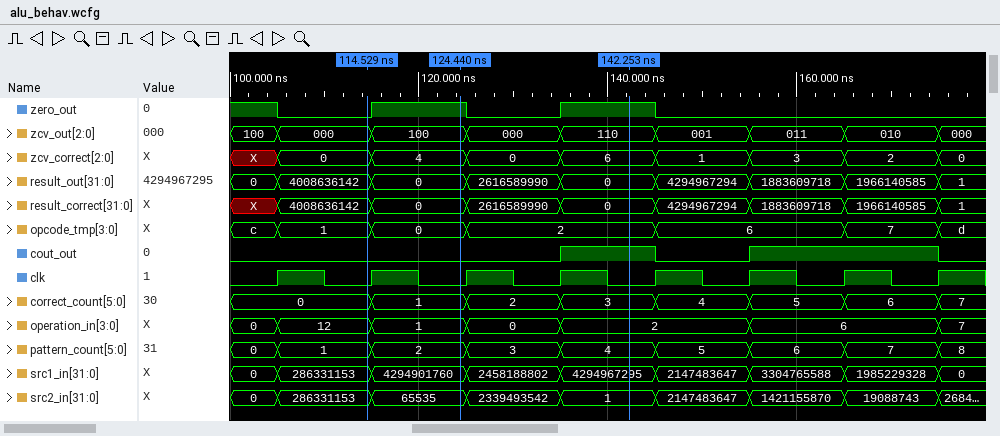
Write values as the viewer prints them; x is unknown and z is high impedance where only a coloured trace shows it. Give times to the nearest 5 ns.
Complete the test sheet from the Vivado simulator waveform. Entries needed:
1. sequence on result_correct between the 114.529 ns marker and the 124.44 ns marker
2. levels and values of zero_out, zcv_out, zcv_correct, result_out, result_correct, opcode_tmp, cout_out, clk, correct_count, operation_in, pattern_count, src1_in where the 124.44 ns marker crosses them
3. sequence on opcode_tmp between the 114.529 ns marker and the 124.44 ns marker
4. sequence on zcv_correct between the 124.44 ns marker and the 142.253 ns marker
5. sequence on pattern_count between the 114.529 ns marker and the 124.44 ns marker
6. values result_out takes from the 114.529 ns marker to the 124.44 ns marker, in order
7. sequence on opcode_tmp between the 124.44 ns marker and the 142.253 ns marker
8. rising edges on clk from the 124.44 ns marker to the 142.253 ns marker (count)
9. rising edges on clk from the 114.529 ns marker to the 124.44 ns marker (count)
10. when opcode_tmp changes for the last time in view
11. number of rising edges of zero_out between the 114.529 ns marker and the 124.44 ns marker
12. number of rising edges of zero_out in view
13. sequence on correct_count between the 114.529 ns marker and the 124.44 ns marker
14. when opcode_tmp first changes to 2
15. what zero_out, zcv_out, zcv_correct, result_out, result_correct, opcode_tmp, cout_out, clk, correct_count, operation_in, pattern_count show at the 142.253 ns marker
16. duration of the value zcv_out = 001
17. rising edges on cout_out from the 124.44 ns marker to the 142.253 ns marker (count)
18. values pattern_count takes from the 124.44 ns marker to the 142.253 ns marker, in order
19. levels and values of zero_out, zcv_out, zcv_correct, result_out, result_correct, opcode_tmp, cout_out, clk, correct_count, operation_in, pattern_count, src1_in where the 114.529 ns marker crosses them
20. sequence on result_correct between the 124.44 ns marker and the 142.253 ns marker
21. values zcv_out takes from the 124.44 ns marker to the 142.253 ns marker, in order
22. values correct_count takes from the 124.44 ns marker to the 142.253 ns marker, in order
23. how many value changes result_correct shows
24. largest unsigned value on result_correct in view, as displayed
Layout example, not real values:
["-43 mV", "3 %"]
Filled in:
["4008636142, 0", "zero_out=1, zcv_out=100, zcv_correct=4, result_out=0, result_correct=0, opcode_tmp=0, cout_out=0, clk=0, correct_count=1, operation_in=1, pattern_count=2, src1_in=4294901760", "1, 0", "4, 0, 6", "1, 2", "4008636142, 0", "0, 2", "2", "1", "175 ns", "1", "2", "0, 1", "125 ns", "zero_out=1, zcv_out=110, zcv_correct=6, result_out=0, result_correct=0, opcode_tmp=2, cout_out=1, clk=0, correct_count=3, operation_in=2, pattern_count=4", "10 ns", "1", "2, 3, 4", "zero_out=0, zcv_out=000, zcv_correct=0, result_out=4008636142, result_correct=4008636142, opcode_tmp=1, cout_out=0, clk=0, correct_count=0, operation_in=12, pattern_count=1, src1_in=286331153", "0, 2616589990, 0", "100, 000, 110", "1, 2, 3", "8", "4294967294"]
